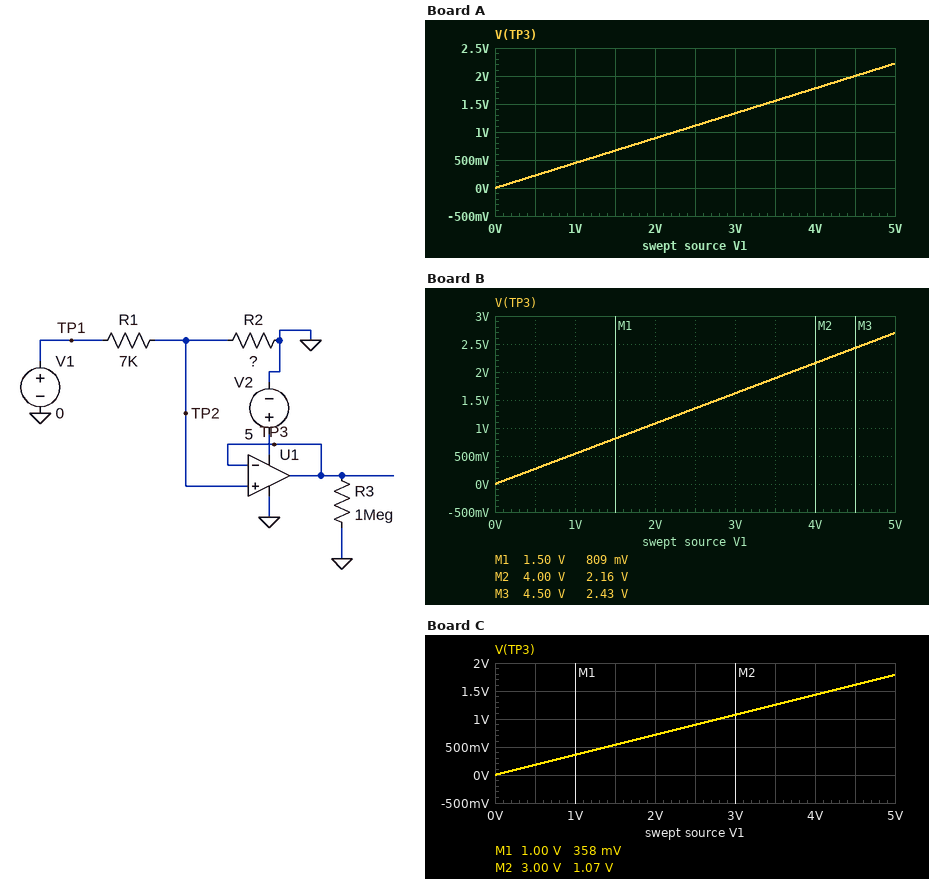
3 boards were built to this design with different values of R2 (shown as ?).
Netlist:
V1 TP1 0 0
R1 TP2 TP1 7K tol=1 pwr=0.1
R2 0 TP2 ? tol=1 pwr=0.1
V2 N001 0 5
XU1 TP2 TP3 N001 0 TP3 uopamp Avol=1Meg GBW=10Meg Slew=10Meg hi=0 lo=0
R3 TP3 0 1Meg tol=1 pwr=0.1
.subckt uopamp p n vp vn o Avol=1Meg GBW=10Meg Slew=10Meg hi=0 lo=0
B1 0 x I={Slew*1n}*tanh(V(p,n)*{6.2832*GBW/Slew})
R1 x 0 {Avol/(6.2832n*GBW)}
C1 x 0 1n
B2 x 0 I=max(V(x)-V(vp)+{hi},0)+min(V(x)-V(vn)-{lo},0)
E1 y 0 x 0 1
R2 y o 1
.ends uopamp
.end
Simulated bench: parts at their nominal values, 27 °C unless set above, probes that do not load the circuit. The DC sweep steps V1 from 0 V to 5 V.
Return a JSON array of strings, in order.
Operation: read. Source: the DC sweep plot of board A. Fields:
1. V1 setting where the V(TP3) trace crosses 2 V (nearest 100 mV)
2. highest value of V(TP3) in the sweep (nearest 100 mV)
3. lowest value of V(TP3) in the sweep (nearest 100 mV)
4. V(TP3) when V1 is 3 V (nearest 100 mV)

["4.5 V", "2.2 V", "0 V", "1.3 V"]
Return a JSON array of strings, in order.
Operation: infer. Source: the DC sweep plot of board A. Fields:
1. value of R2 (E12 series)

["5.6 kΩ"]
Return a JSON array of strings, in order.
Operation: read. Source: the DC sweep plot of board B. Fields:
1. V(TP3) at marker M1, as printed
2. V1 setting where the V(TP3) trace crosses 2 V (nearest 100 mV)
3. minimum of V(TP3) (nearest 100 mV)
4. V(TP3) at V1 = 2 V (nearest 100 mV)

["809 mV", "3.7 V", "0 V", "1.1 V"]
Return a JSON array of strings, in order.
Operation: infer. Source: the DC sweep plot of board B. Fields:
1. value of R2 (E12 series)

["8.2 kΩ"]
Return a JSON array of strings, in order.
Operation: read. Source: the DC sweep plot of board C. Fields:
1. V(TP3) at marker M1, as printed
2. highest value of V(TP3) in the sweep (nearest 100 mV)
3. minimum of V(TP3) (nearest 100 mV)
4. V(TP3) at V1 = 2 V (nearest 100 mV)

["358 mV", "1.8 V", "0 V", "700 mV"]
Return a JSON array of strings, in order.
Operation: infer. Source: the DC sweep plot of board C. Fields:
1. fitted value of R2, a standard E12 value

["3.9 kΩ"]
